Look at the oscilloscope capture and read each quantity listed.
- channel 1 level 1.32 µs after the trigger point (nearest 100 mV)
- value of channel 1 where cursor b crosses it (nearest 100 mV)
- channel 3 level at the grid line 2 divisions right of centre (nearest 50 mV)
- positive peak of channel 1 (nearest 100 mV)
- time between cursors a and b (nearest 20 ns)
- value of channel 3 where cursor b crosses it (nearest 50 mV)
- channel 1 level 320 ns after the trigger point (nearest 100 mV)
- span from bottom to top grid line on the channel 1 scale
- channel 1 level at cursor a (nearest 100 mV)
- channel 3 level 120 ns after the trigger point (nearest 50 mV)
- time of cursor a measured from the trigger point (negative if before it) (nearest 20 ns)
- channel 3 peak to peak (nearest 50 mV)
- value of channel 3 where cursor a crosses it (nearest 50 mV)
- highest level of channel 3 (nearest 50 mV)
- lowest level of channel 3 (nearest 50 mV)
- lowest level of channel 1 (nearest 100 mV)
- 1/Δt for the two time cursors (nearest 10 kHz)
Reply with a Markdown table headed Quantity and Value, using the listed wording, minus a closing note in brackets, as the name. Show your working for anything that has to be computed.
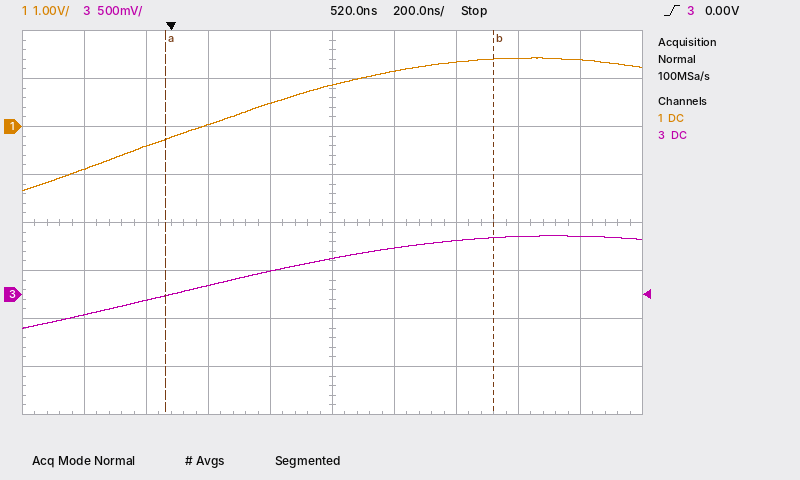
| Quantity | Value |
|---|---|
| channel 1 level 1.32 µs after the trigger point | 1.4 V |
| value of channel 1 where cursor b crosses it | 1.4 V |
| channel 3 level at the grid line 2 divisions right of centre | 550 mV |
| positive peak of channel 1 | 1.4 V |
| time between cursors a and b | 1.06 µs |
| value of channel 3 where cursor b crosses it | 600 mV |
| channel 1 level 320 ns after the trigger point | 500 mV |
| span from bottom to top grid line on the channel 1 scale | 8 V |
| channel 1 level at cursor a | -300 mV |
| channel 3 level 120 ns after the trigger point | 100 mV |
| time of cursor a measured from the trigger point (negative if before it) | -20 ns |
| channel 3 peak to peak | 600 mV − (-350 mV) = 950 mV |
| value of channel 3 where cursor a crosses it | 0 mV |
| highest level of channel 3 | 600 mV |
| lowest level of channel 3 | -350 mV |
| lowest level of channel 1 | -1.3 V |
| 1/Δt for the two time cursors | 1 / 1.06 µs ≈ 940 kHz |
